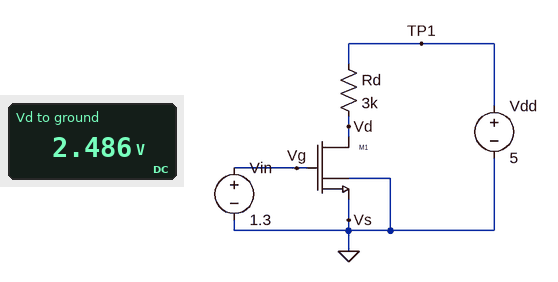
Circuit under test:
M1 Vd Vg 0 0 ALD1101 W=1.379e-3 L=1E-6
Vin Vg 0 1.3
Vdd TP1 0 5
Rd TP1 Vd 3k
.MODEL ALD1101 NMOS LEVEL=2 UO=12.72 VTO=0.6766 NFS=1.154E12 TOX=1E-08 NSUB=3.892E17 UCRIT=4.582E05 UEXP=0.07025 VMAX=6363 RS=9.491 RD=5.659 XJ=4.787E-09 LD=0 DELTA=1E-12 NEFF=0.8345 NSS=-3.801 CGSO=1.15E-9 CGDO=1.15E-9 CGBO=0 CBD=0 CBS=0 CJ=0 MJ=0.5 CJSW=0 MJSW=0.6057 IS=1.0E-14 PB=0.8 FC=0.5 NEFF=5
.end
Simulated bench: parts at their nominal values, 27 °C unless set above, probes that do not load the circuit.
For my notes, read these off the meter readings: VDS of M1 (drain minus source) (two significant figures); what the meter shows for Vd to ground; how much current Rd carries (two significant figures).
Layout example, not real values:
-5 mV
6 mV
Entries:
2.5 V
2.486 V
840 µA
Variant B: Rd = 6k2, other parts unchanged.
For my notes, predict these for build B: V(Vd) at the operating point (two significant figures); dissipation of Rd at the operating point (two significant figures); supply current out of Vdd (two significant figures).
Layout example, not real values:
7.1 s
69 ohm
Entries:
330 mV
3.5 mW
750 µA
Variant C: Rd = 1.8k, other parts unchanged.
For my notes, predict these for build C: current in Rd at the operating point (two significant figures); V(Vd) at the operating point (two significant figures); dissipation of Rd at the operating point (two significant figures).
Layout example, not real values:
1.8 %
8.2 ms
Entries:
850 µA
3.5 V
1.3 mW
